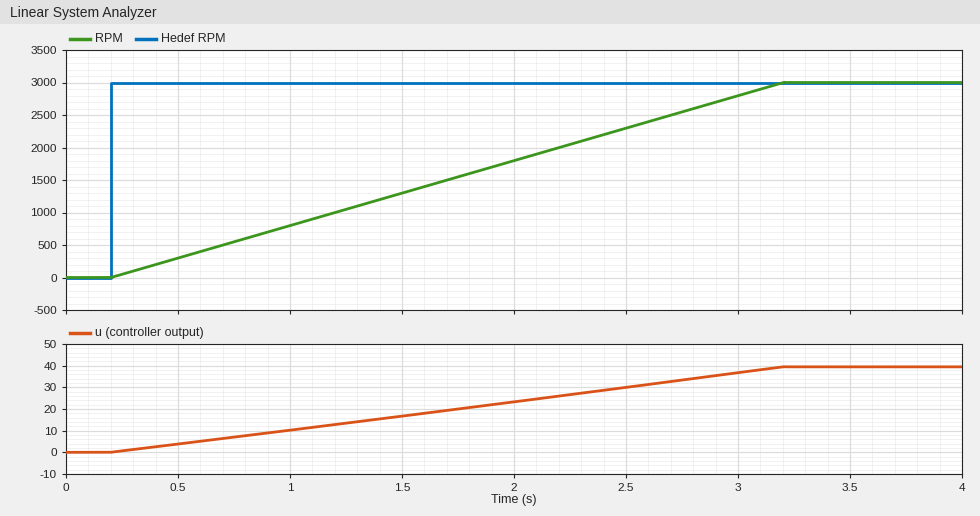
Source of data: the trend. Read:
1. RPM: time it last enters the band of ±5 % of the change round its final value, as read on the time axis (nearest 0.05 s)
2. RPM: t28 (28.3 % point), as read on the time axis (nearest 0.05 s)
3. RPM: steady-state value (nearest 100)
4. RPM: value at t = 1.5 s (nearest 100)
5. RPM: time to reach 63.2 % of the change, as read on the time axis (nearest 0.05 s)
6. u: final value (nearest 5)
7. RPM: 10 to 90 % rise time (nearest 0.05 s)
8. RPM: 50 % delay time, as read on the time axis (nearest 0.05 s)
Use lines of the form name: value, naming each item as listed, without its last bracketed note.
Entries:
RPM: time it last enters the band of ±5 % of the change round its final value, as read on the time axis: 3.05 s
RPM: t28 (28.3 % point), as read on the time axis: 1.05 s
RPM: steady-state value: 3000
RPM: value at t = 1.5 s: 1300
RPM: time to reach 63.2 % of the change, as read on the time axis: 2.10 s
u: final value: 40
RPM: 10 to 90 % rise time: 2.40 s
RPM: 50 % delay time, as read on the time axis: 1.70 s
